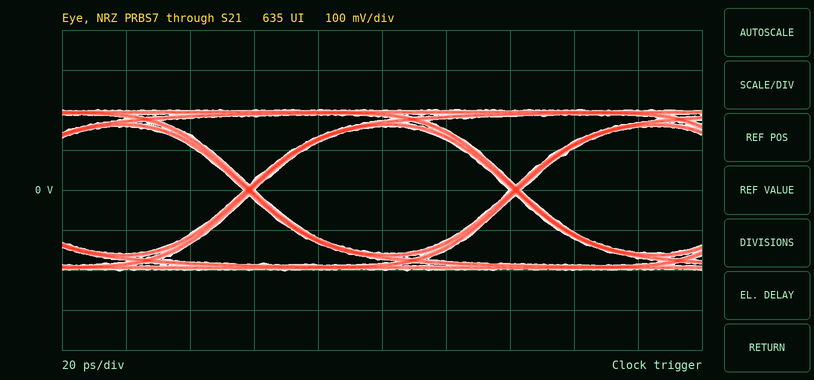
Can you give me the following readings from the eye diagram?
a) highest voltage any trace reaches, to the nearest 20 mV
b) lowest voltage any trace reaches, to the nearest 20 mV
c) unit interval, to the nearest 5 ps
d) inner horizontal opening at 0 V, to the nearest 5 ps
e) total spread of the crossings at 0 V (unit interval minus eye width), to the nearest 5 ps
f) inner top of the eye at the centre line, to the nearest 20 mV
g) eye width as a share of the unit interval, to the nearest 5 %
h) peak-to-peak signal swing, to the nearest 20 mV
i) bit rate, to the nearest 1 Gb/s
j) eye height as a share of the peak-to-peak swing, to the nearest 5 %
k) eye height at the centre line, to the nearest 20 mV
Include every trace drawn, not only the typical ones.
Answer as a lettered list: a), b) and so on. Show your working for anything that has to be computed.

a) 200 mV
b) -200 mV
c) 85 ps
d) 80 ps
e) 5 ps
f) 160 mV
g) 80 ps / 85 ps ≈ 94.1 %, so 95 % to the nearest 5 %
h) 400 mV
i) 12 Gb/s
j) 320 mV / 400 mV ≈ 80 %
k) 320 mV
